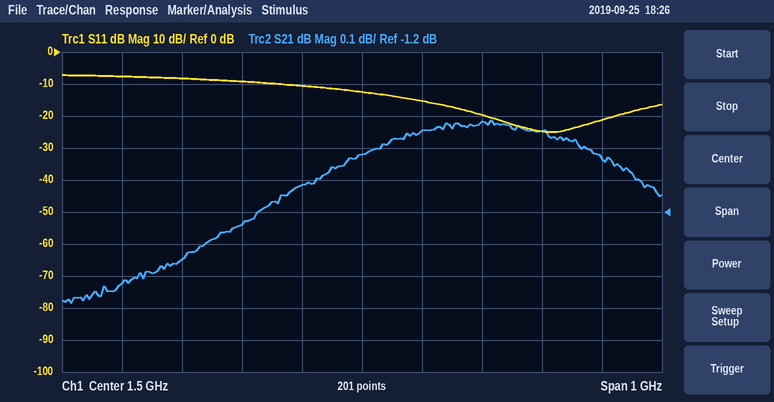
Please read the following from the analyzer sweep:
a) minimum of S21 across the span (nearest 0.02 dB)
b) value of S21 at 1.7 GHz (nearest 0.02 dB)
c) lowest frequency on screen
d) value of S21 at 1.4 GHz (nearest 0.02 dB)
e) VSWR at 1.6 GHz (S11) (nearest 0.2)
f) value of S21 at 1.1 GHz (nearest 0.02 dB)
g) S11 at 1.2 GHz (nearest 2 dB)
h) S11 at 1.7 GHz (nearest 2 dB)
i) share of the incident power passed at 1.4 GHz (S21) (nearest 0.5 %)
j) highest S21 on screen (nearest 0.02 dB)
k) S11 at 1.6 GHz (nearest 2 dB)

-1.48 dB
-0.92 dB
1 GHz
-1.12 dB
1.4
-1.42 dB
-8 dB
-20 dB
77.5 %
-0.92 dB
-16 dB
